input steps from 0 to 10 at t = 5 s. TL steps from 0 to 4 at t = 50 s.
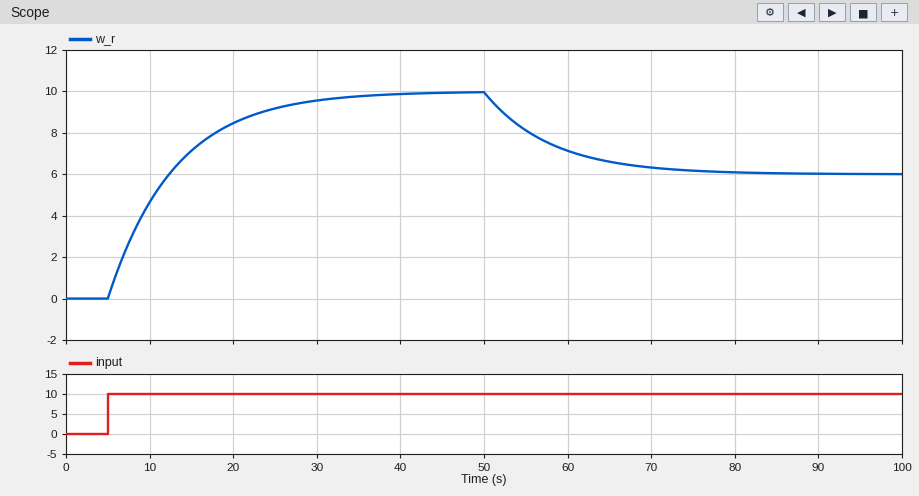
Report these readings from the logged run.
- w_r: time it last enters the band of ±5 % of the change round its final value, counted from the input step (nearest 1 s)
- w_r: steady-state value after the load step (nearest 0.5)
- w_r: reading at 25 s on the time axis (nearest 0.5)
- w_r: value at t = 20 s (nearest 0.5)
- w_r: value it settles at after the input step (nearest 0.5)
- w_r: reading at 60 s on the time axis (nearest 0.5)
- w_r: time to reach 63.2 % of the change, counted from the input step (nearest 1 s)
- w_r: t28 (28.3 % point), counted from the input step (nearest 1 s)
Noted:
24 s
6.0
9.0
8.5
10.0
7.0
8 s
3 s
